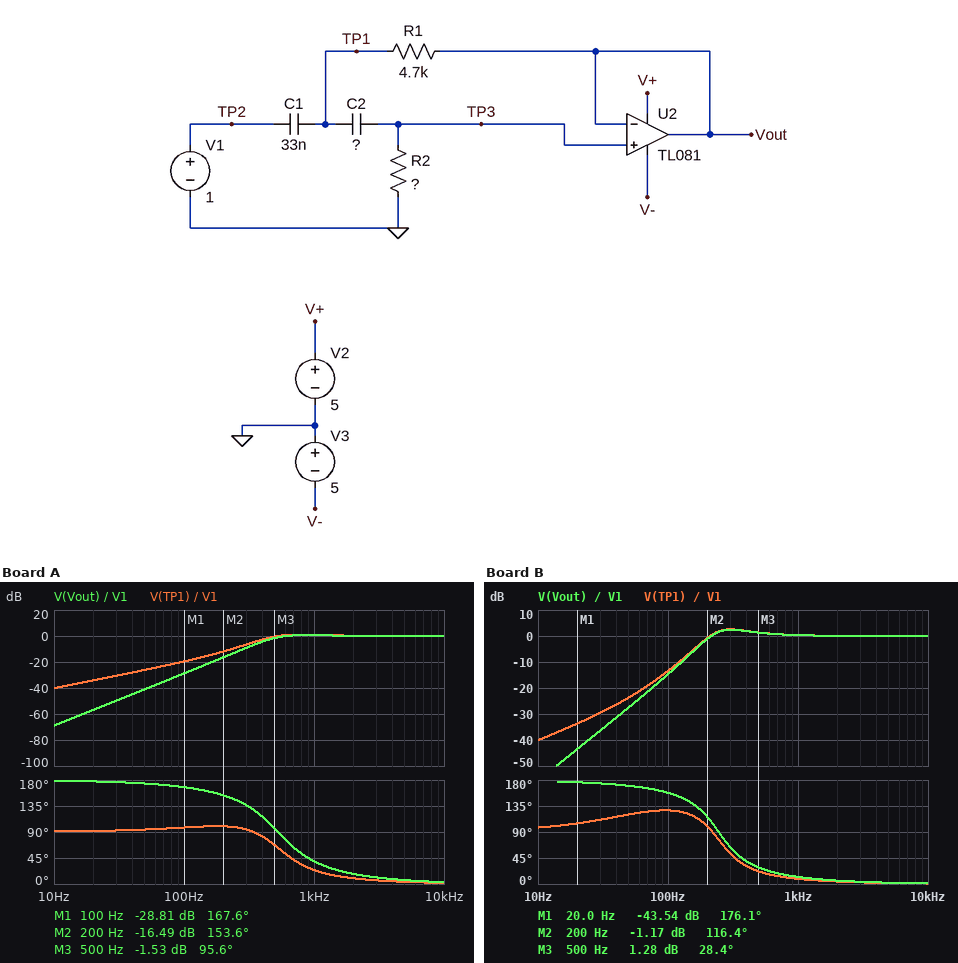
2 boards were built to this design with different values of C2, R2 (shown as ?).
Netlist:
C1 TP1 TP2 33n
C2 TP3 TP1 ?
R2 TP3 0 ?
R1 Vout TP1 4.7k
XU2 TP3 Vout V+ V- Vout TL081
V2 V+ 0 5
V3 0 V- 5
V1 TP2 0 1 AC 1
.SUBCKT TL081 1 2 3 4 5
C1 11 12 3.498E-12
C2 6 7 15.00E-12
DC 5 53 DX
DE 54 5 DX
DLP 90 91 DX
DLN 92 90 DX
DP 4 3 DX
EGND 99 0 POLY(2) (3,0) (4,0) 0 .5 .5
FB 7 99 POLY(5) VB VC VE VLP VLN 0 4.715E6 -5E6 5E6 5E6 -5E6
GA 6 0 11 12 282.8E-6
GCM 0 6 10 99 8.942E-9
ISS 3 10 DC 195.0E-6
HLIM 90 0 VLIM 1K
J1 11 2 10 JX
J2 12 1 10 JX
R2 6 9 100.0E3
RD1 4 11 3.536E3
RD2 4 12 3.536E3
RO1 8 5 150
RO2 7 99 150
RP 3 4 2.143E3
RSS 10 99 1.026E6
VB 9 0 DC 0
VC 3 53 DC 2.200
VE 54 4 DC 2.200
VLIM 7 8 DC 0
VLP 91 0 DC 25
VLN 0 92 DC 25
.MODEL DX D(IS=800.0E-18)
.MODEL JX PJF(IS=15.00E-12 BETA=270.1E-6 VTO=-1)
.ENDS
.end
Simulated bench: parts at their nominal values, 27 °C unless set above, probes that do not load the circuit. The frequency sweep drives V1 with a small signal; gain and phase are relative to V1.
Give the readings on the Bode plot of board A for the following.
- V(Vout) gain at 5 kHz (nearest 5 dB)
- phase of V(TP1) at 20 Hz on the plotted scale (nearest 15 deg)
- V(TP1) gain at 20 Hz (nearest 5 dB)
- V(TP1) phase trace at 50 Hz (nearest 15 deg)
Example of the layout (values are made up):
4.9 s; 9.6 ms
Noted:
0 dB; 90 deg; -35 dB; 90 deg
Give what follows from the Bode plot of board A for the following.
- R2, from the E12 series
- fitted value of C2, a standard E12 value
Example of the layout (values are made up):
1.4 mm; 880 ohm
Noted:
15 kΩ; 39 nF
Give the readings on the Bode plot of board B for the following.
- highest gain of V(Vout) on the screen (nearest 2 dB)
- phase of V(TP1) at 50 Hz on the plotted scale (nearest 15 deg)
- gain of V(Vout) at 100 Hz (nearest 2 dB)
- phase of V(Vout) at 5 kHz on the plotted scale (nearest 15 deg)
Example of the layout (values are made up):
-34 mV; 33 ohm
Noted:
2 dB; 120 deg; -14 dB; 0 deg
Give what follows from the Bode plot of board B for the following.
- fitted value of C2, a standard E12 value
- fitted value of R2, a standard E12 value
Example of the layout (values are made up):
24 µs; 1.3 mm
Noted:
82 nF; 33 kΩ
